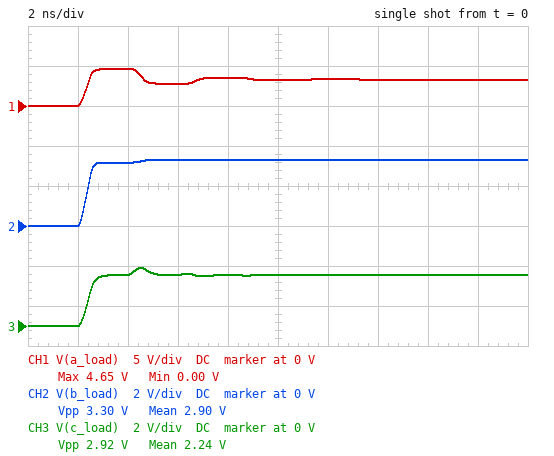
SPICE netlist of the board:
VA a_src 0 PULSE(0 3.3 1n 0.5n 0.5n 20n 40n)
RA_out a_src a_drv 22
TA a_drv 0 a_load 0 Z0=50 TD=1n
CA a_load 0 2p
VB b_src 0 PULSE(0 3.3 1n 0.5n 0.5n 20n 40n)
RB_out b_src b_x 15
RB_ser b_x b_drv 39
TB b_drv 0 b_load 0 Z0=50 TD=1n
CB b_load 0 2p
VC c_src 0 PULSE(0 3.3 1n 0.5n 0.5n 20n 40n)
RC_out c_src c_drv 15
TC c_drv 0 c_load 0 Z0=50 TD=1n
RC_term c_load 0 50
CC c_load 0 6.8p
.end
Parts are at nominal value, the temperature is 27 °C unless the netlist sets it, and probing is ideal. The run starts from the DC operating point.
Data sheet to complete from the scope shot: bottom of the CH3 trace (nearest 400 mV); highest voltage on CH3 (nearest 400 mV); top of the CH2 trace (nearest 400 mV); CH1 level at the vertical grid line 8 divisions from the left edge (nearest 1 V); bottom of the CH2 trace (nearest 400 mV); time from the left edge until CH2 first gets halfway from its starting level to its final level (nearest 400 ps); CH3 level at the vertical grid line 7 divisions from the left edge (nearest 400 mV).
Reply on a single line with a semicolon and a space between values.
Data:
0 V; 2.8 V; 3.2 V; 3 V; 0 V; 2.4 ns; 2.4 V
